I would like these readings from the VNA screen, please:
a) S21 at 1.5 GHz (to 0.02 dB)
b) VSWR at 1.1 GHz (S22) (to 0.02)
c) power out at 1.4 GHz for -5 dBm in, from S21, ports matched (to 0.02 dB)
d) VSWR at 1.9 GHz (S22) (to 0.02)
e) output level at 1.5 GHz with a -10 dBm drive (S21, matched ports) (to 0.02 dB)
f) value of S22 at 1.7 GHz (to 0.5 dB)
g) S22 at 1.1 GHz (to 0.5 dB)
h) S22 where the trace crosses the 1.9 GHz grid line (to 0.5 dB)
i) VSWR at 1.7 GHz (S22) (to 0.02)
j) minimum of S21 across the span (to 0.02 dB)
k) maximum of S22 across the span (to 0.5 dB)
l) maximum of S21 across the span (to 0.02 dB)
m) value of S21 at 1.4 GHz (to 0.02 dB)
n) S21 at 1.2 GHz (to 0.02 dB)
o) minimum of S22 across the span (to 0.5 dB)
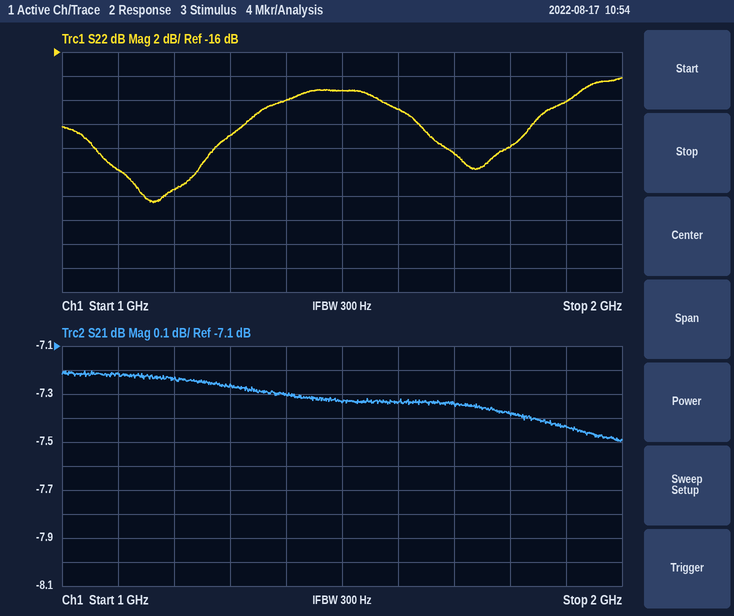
-7.34 dB
1.10
-12.30 dBm
1.22
-17.34 dBm
-24.5 dB
-26.0 dB
-20.0 dB
1.12
-7.50 dB
-18.0 dB
-7.20 dB
-7.30 dB
-7.24 dB
-28.5 dB
